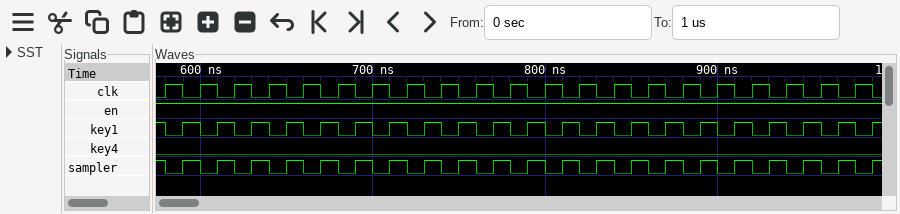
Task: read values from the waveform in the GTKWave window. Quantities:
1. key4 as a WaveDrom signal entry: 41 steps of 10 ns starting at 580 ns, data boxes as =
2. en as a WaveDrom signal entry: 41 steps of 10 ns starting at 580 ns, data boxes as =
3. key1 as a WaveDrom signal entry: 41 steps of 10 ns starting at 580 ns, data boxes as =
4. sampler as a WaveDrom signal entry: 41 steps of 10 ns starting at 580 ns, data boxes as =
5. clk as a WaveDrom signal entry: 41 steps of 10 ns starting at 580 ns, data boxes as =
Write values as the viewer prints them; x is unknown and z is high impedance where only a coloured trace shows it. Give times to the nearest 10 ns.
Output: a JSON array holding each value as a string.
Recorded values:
["{name: 'key4', wave: '0........................................'}", "{name: 'en', wave: '1........................................'}", "{name: 'key1', wave: '01010101010101010101010101010101010101010'}", "{name: 'sampler', wave: '01010101010101010101010101010101010101010'}", "{name: 'clk', wave: '10101010101010101010101010101010101010101'}"]
